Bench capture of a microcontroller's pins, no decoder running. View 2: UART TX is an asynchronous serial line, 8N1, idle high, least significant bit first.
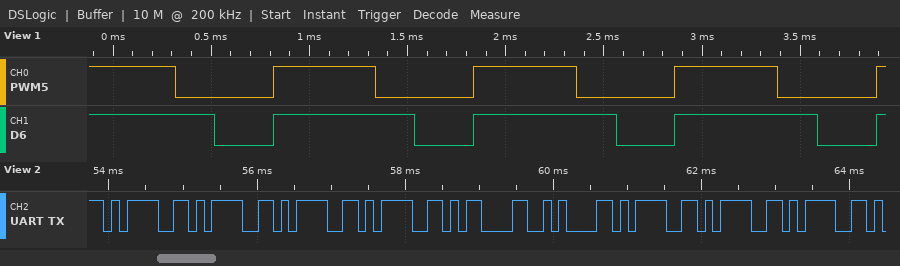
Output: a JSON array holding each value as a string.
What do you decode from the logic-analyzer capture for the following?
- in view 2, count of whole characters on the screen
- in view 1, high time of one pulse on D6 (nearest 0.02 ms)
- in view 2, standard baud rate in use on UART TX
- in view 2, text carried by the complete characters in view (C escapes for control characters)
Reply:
["9", "0.72 ms", "9600 baud", "\"====\\r\\n===\""]
